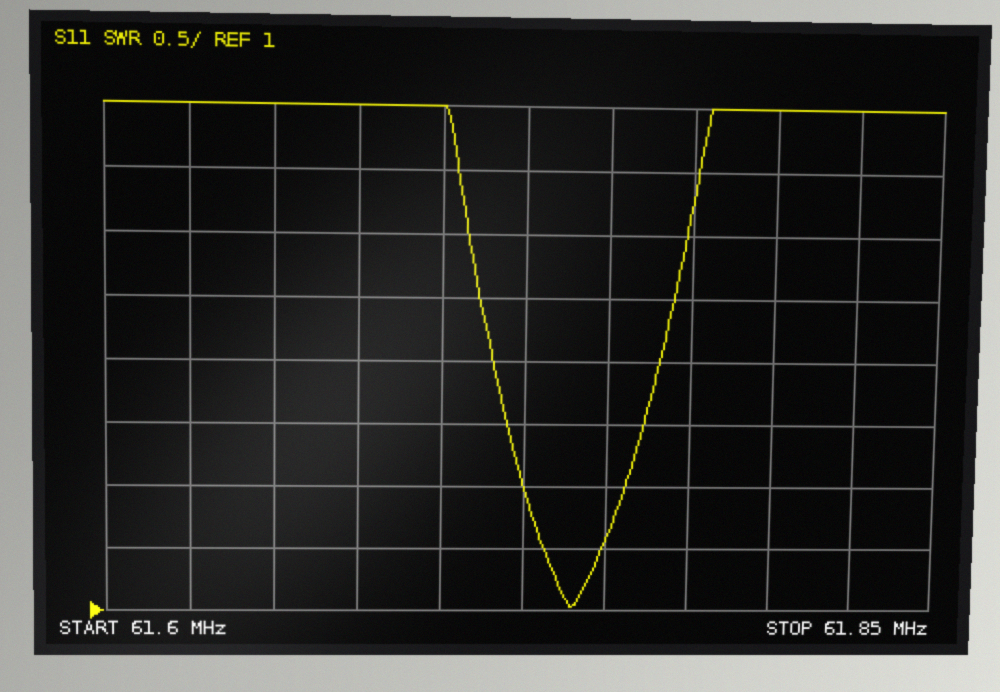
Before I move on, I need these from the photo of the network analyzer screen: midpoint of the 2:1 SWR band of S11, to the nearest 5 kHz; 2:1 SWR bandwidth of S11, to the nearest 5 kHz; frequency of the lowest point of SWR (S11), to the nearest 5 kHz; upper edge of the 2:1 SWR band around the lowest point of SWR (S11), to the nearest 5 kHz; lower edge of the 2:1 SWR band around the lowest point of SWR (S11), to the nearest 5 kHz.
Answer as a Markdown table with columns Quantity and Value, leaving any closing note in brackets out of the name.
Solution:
| Quantity | Value |
|---|---|
| midpoint of the 2:1 SWR band of S11, to the nearest 5 kHz | 61.740 MHz |
| 2:1 SWR bandwidth of S11, to the nearest 5 kHz | 30 kHz |
| frequency of the lowest point of SWR (S11), to the nearest 5 kHz | 61.740 MHz |
| upper edge of the 2:1 SWR band around the lowest point of SWR (S11), to the nearest 5 kHz | 61.755 MHz |
| lower edge of the 2:1 SWR band around the lowest point of SWR (S11), to the nearest 5 kHz | 61.725 MHz |
